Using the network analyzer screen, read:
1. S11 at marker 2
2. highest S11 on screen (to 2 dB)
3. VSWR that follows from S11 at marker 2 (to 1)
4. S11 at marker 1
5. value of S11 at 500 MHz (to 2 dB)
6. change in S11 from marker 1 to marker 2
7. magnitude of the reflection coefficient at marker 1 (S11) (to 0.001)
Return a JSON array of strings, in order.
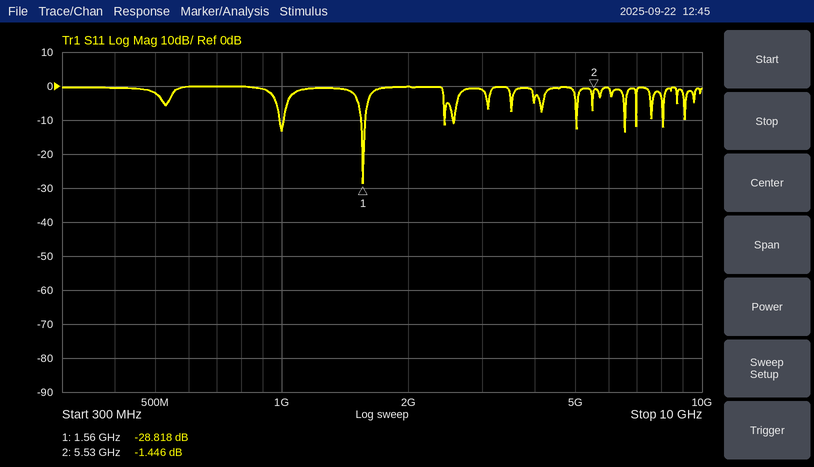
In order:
["-1.446 dB", "0 dB", "12", "-28.818 dB", "-2 dB", "27.372 dB", "0.036"]
